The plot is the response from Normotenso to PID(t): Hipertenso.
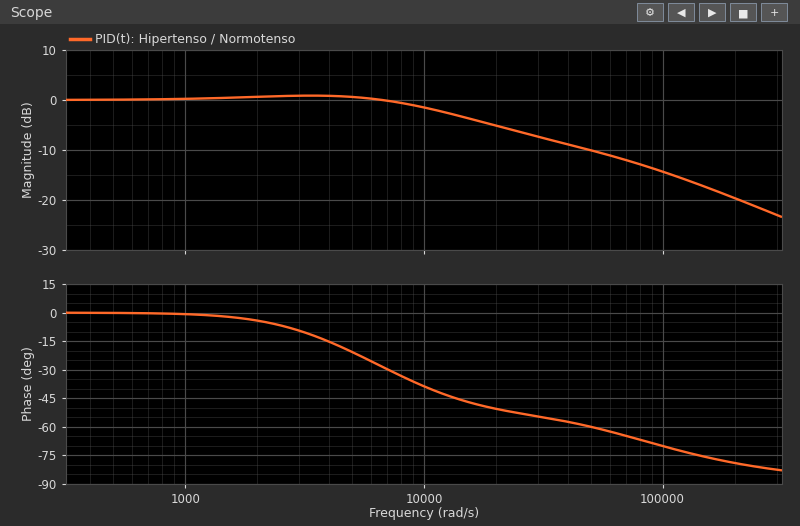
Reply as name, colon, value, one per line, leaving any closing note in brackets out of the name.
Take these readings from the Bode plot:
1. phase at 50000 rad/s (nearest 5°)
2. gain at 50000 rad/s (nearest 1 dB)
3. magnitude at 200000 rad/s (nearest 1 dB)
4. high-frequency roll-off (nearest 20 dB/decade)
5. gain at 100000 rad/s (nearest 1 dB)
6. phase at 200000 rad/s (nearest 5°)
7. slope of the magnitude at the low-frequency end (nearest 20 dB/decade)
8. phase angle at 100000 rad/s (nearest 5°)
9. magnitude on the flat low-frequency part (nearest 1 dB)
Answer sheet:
phase at 50000 rad/s: -60°
gain at 50000 rad/s: -10 dB
magnitude at 200000 rad/s: -20 dB
high-frequency roll-off: -20 dB/decade
gain at 100000 rad/s: -14 dB
phase at 200000 rad/s: -80°
slope of the magnitude at the low-frequency end: 0 dB/decade
phase angle at 100000 rad/s: -70°
magnitude on the flat low-frequency part: 0 dB
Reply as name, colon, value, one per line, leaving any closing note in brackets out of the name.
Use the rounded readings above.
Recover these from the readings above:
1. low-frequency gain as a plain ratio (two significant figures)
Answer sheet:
low-frequency gain as a plain ratio: 1.0
